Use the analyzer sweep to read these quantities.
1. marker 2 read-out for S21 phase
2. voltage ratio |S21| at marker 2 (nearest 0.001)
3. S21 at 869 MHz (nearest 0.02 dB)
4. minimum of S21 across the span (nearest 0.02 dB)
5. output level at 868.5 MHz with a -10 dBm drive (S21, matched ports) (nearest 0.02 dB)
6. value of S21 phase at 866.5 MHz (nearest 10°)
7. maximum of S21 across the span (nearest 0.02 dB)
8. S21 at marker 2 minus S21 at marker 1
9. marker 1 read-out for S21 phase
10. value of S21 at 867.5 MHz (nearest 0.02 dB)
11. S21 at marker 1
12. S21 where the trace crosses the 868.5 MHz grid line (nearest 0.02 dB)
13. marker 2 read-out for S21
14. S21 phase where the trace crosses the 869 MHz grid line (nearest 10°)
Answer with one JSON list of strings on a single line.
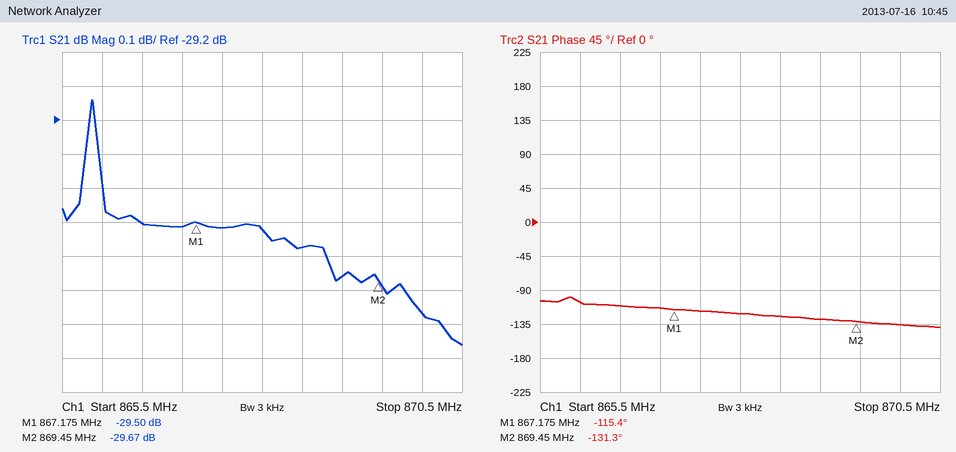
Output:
["-131.3°", "0.033", "-29.66 dB", "-29.86 dB", "-39.58 dBm", "-110°", "-29.14 dB", "-0.17 dB", "-115.4°", "-29.52 dB", "-29.50 dB", "-29.58 dB", "-29.67 dB", "-130°"]
